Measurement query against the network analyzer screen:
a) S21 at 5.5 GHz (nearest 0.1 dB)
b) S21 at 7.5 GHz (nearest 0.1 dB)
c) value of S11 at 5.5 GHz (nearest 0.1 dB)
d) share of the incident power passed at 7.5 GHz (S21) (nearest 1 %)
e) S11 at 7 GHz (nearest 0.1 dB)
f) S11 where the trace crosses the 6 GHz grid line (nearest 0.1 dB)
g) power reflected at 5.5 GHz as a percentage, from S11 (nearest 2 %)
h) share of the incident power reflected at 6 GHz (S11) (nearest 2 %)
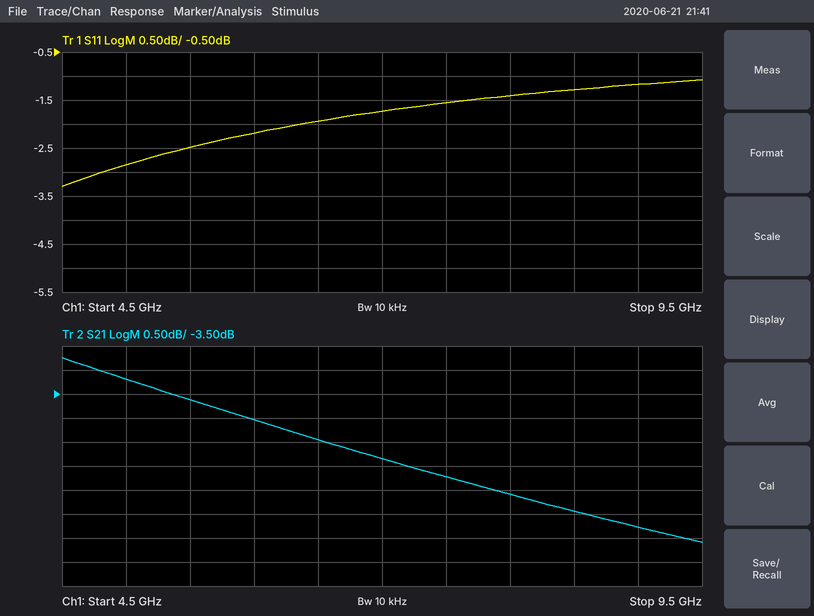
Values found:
-3.6 dB
-5.2 dB
-2.5 dB
30 %
-1.7 dB
-2.2 dB
56 %
60 %
